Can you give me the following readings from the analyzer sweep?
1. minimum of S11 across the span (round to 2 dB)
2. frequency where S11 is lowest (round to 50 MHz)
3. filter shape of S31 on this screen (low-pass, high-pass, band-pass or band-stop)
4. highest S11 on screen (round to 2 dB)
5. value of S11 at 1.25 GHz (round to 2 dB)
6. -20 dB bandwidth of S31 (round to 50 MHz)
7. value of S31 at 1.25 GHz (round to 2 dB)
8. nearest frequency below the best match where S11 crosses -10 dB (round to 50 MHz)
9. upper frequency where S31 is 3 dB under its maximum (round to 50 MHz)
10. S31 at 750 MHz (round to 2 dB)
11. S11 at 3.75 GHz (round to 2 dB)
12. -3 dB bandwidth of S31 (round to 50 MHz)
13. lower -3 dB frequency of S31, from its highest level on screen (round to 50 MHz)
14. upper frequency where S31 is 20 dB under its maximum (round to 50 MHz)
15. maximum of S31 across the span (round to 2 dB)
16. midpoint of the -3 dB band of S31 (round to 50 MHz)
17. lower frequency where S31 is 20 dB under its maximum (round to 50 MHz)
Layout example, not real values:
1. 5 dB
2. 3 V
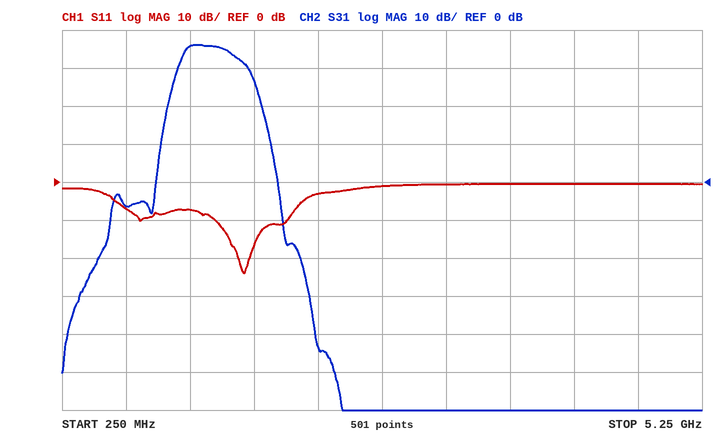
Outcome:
1. -24 dB
2. 1.65 GHz
3. band-pass
4. 0 dB
5. -8 dB
6. 800 MHz
7. 36 dB
8. 1.45 GHz
9. 1.60 GHz
10. -6 dB
11. 0 dB
12. 400 MHz
13. 1.20 GHz
14. 1.85 GHz
15. 36 dB
16. 1.40 GHz
17. 1.05 GHz
